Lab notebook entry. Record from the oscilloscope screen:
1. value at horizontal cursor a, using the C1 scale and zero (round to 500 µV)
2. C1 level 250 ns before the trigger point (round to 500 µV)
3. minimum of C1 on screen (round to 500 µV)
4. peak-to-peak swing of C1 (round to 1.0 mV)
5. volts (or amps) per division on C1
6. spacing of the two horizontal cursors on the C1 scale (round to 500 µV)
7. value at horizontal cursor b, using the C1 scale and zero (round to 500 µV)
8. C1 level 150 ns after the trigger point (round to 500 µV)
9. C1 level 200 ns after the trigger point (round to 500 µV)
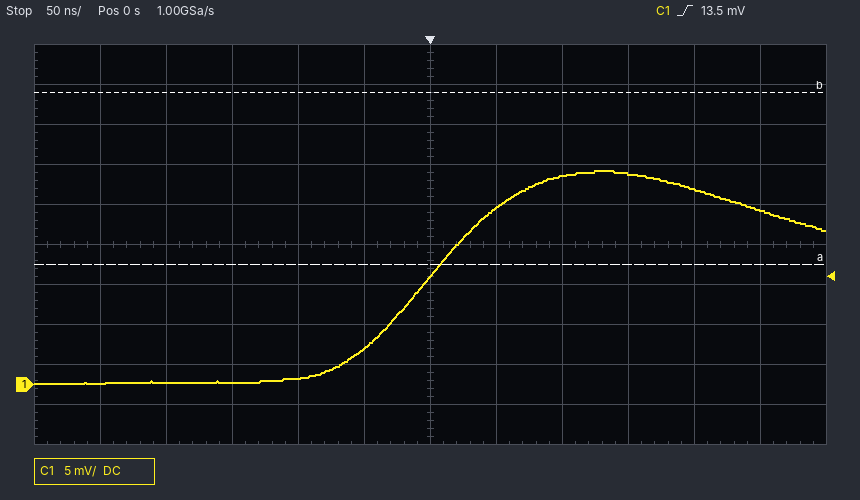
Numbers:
15.0 mV
0.0 mV
0.0 mV
27.0 mV
5 mV
21.5 mV
36.5 mV
26.5 mV
24.5 mV
